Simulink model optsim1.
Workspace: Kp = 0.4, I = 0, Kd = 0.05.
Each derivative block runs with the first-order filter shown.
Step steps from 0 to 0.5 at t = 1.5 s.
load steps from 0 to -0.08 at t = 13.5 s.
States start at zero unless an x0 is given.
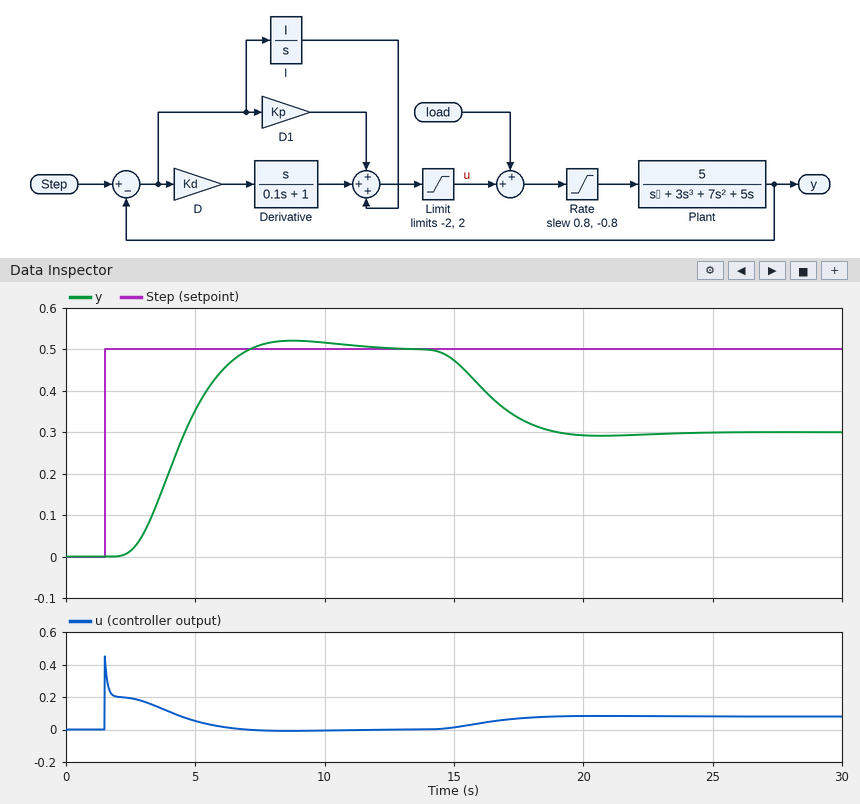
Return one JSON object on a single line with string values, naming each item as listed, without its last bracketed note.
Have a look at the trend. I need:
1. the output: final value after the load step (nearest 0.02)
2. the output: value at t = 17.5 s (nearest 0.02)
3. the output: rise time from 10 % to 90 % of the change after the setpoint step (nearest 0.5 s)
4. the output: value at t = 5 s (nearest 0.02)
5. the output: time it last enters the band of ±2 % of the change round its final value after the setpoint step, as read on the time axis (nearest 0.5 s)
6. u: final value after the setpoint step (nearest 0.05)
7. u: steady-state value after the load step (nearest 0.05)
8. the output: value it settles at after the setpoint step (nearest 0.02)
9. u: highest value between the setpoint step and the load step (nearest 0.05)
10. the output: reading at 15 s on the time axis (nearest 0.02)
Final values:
{"the output: final value after the load step": "0.30", "the output: value at t = 17.5 s": "0.34", "the output: rise time from 10 % to 90 % of the change after the setpoint step": "3.0 s", "the output: value at t = 5 s": "0.36", "the output: time it last enters the band of ±2 % of the change round its final value after the setpoint step, as read on the time axis": "11.0 s", "u: final value after the setpoint step": "0.00", "u: steady-state value after the load step": "0.10", "the output: value it settles at after the setpoint step": "0.50", "u: highest value between the setpoint step and the load step": "0.45", "the output: reading at 15 s on the time axis": "0.48"}
